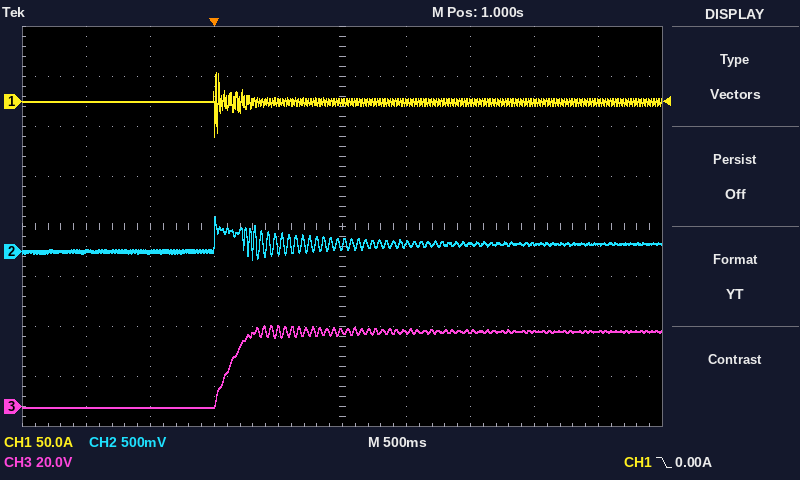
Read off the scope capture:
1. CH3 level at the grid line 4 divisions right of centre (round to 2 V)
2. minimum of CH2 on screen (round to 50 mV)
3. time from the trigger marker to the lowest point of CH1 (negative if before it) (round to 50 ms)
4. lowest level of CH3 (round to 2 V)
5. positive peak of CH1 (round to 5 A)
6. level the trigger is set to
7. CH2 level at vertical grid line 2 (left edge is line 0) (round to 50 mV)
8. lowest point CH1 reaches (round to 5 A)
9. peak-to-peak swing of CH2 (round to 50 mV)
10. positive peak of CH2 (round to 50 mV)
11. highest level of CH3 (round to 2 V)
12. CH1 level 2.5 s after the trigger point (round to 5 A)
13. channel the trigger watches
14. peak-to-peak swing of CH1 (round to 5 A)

30 V
-100 mV
0 ms
0 V
30 A
0.00 A
0 mV
-35 A
450 mV
350 mV
32 V
0 A
CH1
65 A
